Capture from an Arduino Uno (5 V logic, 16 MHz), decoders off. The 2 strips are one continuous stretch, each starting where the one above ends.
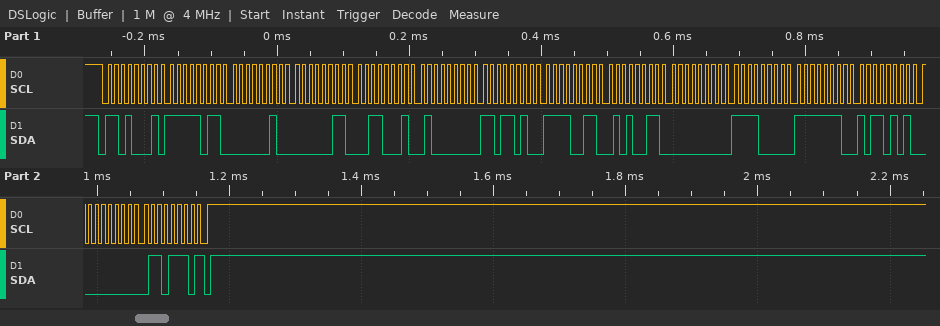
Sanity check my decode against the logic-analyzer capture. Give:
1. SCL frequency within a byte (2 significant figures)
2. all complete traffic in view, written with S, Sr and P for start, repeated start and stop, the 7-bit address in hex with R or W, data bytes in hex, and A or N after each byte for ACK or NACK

100 kHz
S 68R A FB A 02 A 03 A 31 A 40 A DA A F3 A 53 A 00 A F0 A FE A B5 A 00 A 6E N P
